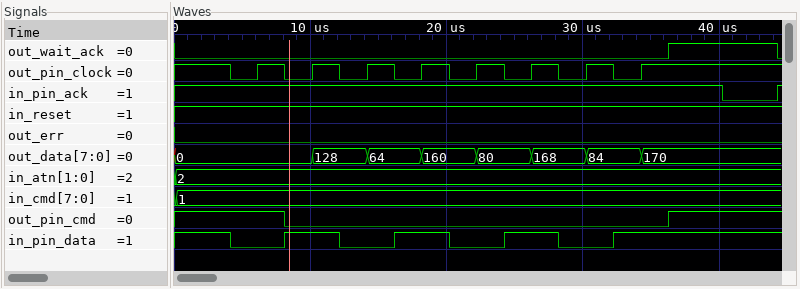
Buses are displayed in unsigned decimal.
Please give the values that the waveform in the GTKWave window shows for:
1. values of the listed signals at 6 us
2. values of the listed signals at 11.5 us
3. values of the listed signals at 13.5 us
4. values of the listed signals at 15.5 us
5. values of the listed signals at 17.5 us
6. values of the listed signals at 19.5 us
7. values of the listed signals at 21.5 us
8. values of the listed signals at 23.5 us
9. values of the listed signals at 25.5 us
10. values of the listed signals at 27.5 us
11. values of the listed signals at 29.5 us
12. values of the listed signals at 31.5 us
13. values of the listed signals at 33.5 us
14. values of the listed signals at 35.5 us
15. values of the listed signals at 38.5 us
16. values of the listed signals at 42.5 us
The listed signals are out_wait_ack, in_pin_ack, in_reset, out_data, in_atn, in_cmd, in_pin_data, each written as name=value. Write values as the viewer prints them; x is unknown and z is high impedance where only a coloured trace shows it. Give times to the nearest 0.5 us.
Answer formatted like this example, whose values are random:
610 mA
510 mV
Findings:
out_wait_ack=0, in_pin_ack=1, in_reset=1, out_data=0, in_atn=2, in_cmd=1, in_pin_data=0
out_wait_ack=0, in_pin_ack=1, in_reset=1, out_data=128, in_atn=2, in_cmd=1, in_pin_data=1
out_wait_ack=0, in_pin_ack=1, in_reset=1, out_data=128, in_atn=2, in_cmd=1, in_pin_data=0
out_wait_ack=0, in_pin_ack=1, in_reset=1, out_data=64, in_atn=2, in_cmd=1, in_pin_data=0
out_wait_ack=0, in_pin_ack=1, in_reset=1, out_data=64, in_atn=2, in_cmd=1, in_pin_data=1
out_wait_ack=0, in_pin_ack=1, in_reset=1, out_data=160, in_atn=2, in_cmd=1, in_pin_data=1
out_wait_ack=0, in_pin_ack=1, in_reset=1, out_data=160, in_atn=2, in_cmd=1, in_pin_data=0
out_wait_ack=0, in_pin_ack=1, in_reset=1, out_data=80, in_atn=2, in_cmd=1, in_pin_data=0
out_wait_ack=0, in_pin_ack=1, in_reset=1, out_data=80, in_atn=2, in_cmd=1, in_pin_data=1
out_wait_ack=0, in_pin_ack=1, in_reset=1, out_data=168, in_atn=2, in_cmd=1, in_pin_data=1
out_wait_ack=0, in_pin_ack=1, in_reset=1, out_data=168, in_atn=2, in_cmd=1, in_pin_data=0
out_wait_ack=0, in_pin_ack=1, in_reset=1, out_data=84, in_atn=2, in_cmd=1, in_pin_data=0
out_wait_ack=0, in_pin_ack=1, in_reset=1, out_data=84, in_atn=2, in_cmd=1, in_pin_data=1
out_wait_ack=0, in_pin_ack=1, in_reset=1, out_data=170, in_atn=2, in_cmd=1, in_pin_data=1
out_wait_ack=1, in_pin_ack=1, in_reset=1, out_data=170, in_atn=2, in_cmd=1, in_pin_data=1
out_wait_ack=1, in_pin_ack=0, in_reset=1, out_data=170, in_atn=2, in_cmd=1, in_pin_data=1
